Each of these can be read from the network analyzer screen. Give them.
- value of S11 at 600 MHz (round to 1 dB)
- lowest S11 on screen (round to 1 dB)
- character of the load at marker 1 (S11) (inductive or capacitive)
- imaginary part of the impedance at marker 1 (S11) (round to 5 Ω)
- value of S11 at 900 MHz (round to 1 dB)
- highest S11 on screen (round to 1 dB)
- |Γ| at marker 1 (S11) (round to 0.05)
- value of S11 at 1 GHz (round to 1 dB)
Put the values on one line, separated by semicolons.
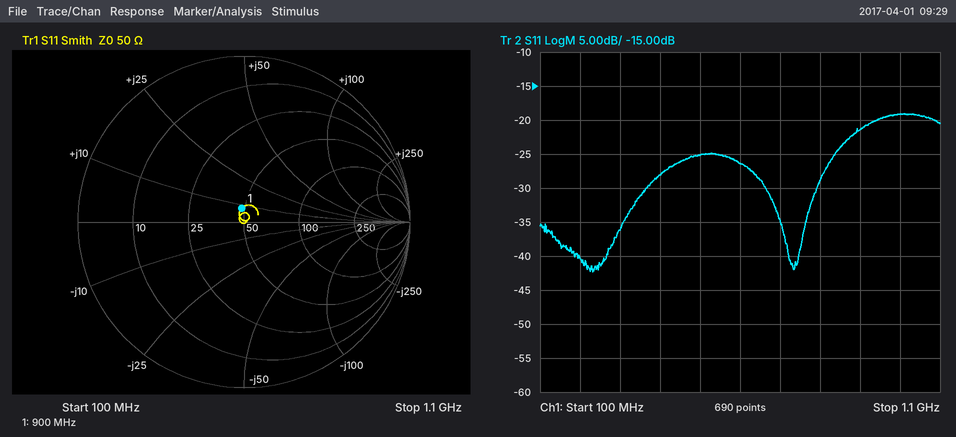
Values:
-26 dB; -42 dB; inductive; +10 Ω; -21 dB; -19 dB; 0.10; -19 dB
